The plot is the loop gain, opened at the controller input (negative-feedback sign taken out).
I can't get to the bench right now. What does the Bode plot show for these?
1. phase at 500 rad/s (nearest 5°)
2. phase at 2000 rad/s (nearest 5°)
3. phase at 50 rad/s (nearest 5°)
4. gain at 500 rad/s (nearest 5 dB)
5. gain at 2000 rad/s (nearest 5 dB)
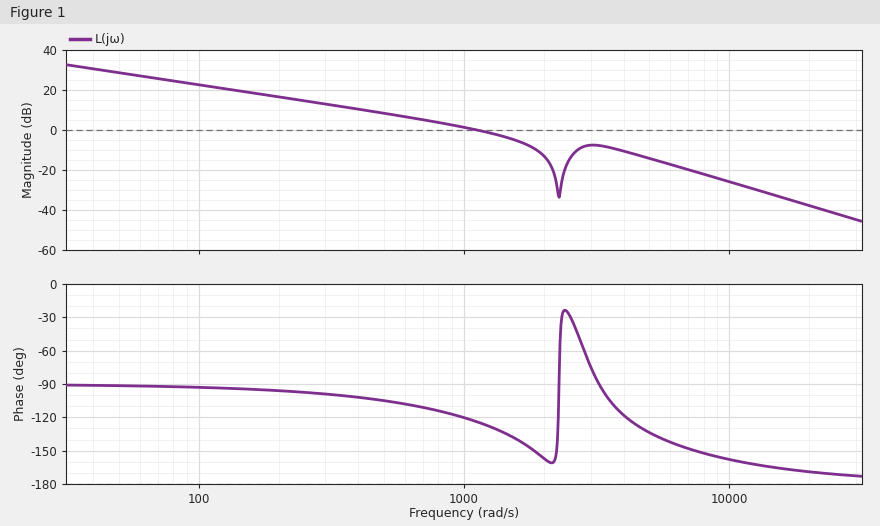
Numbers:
-105°
-155°
-90°
10 dB
-15 dB
